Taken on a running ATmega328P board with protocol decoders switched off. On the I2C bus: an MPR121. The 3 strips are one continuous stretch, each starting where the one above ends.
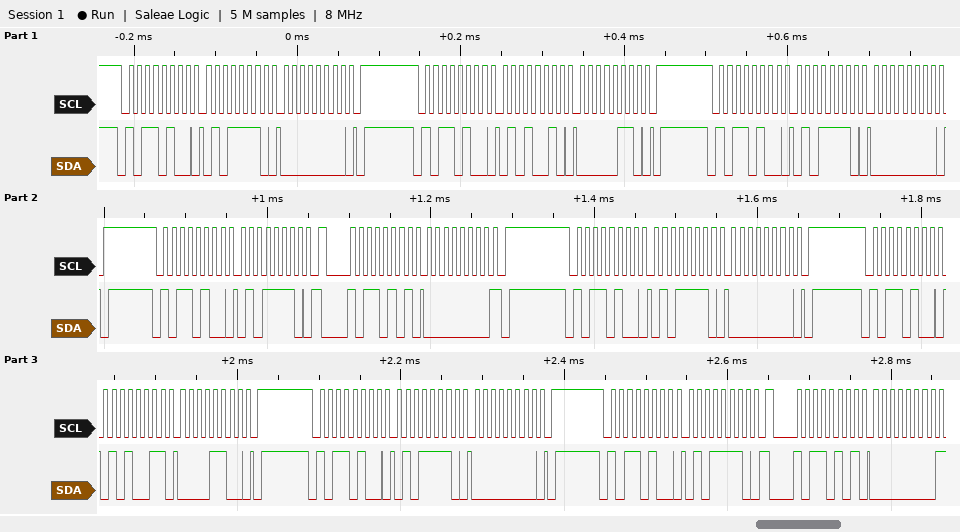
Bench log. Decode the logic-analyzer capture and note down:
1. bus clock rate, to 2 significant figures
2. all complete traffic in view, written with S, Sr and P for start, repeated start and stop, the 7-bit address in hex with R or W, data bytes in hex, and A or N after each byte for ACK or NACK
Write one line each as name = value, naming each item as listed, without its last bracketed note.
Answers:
bus clock rate, to 2 significant figures = 100 kHz
all complete traffic in view, written with S, Sr and P for start, repeated start and stop, the 7-bit address in hex with R or W, data bytes in hex, and A or N after each byte for ACK or NACK = S 5AW A 5E A 00 A P S 5AW A 52 A 06 A P S 5AW A 5E A 00 A P S 5AW A 5E A Sr 5AR A 00 N P S 5AW A 5E A 00 A P S 5AW A 53 A 0C A P S 5AW A 5E A 00 A P S 5AW A 5E A Sr 5AR A 00 N
